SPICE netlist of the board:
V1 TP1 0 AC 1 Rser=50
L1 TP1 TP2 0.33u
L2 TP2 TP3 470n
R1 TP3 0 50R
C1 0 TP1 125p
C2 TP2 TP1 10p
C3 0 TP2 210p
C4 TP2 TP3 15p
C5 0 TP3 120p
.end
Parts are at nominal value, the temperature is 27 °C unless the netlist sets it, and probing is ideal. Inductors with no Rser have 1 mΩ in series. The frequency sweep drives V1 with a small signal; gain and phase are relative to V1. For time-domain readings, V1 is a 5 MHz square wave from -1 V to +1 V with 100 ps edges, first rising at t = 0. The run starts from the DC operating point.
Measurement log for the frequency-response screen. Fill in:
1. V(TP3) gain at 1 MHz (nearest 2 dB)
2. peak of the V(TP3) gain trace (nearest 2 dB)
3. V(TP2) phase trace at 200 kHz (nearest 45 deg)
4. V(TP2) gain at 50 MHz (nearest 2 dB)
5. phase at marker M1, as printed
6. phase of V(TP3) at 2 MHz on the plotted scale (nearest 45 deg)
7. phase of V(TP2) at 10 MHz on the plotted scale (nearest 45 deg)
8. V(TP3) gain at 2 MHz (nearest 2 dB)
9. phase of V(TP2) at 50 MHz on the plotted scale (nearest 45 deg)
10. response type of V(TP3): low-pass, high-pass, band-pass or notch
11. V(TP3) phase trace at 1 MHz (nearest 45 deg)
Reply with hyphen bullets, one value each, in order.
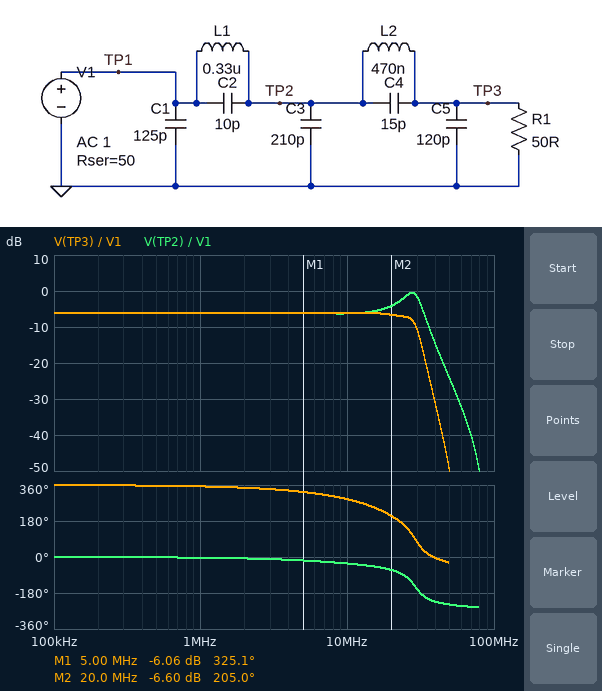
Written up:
- -6 dB
- -6 dB
- 0 deg
- -24 dB
- 325.1 deg
- 360 deg
- -45 deg
- -6 dB
- -225 deg
- low-pass
- 360 deg
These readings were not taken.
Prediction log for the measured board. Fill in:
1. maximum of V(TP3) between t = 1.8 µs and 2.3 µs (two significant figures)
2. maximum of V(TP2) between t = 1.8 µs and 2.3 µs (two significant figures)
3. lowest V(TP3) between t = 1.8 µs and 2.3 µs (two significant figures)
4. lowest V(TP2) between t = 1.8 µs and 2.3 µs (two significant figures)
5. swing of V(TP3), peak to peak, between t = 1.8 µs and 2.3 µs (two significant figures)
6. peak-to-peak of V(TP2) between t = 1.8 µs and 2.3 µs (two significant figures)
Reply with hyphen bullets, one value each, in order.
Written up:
- 650 mV
- 750 mV
- -650 mV
- -750 mV
- 1.3 V
- 1.5 V
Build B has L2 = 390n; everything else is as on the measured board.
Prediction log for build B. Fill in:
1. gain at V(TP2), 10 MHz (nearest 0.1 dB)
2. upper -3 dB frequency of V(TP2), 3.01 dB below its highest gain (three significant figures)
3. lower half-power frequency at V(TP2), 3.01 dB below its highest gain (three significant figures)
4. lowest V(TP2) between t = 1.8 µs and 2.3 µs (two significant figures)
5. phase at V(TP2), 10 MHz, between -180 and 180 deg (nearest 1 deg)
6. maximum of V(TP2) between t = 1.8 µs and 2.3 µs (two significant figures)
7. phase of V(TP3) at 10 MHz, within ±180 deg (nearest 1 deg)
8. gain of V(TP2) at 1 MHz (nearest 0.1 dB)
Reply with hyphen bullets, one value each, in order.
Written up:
- -6.5 dB
- 32.6 MHz
- 23.1 MHz
- -680 mV
- -35 deg
- 680 mV
- -67 deg
- -6.0 dB
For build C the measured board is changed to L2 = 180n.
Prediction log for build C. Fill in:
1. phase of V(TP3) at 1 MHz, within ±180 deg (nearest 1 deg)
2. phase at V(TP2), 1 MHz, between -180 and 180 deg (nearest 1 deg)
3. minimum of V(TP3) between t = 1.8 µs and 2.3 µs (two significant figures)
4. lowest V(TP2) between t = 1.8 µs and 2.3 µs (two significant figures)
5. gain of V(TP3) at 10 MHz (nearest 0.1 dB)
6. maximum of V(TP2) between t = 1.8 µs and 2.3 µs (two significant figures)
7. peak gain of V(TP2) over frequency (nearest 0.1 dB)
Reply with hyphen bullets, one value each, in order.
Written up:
- -6 deg
- -5 deg
- -620 mV
- -520 mV
- -6.4 dB
- 520 mV
- -6.0 dB
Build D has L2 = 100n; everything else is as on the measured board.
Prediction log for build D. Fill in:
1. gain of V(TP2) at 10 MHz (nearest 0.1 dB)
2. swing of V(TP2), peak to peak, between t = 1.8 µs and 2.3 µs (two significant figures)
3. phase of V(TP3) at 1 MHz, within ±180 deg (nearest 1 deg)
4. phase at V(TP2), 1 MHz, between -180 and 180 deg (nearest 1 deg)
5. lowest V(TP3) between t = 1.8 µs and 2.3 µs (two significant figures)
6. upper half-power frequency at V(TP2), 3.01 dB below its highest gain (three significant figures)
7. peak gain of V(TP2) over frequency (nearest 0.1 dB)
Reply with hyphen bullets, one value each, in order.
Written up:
- -6.9 dB
- 1.0 V
- -6 deg
- -5 deg
- -540 mV
- 22.9 MHz
- -6.0 dB
